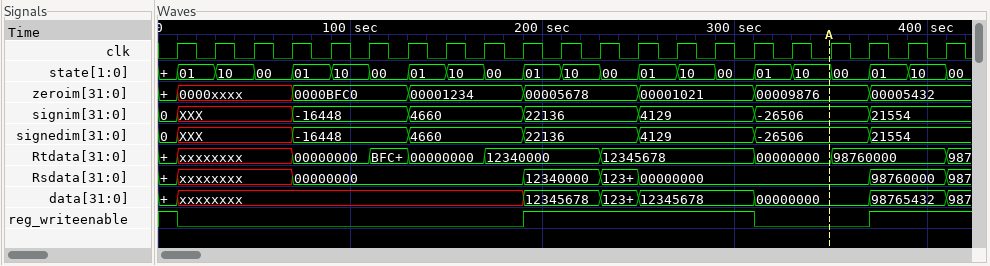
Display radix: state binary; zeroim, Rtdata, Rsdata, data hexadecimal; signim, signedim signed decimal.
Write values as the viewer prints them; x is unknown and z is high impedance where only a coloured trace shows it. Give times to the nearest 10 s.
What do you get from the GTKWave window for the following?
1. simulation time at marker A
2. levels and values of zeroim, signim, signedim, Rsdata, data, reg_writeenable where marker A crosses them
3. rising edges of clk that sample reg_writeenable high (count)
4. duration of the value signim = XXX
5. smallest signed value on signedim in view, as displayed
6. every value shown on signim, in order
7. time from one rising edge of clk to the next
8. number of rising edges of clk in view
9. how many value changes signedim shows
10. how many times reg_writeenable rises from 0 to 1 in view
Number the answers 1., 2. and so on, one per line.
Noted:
1. 350 s
2. zeroim=00009876, signim=-26506, signedim=-26506, Rsdata=00000000, data=00000000, reg_writeenable=0
3. 9
4. 60 s
5. -26506
6. 0, XXX, -16448, 4660, 22136, 4129, -26506, 21554
7. 20 s
8. 21
9. 7
10. 2
